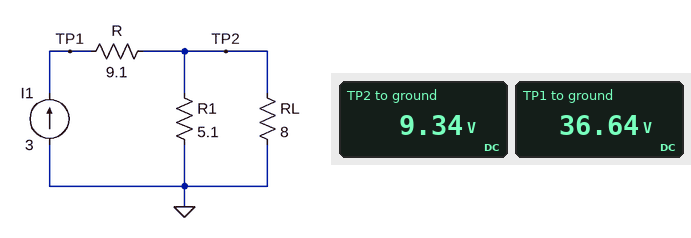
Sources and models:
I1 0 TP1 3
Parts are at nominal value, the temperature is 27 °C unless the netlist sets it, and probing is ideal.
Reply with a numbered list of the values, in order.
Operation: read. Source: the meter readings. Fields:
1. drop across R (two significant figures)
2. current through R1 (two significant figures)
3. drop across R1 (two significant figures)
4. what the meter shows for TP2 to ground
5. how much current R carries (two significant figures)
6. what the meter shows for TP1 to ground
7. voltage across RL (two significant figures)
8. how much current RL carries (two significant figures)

1. 27 V
2. 1.8 A
3. 9.3 V
4. 9.34 V
5. 3.0 A
6. 36.64 V
7. 9.3 V
8. 1.2 A
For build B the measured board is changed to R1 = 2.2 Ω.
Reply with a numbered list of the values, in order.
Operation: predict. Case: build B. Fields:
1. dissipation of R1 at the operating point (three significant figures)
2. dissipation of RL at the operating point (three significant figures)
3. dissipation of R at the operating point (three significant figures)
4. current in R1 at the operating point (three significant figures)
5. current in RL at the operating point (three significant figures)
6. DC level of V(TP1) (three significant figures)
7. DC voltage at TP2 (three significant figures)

1. 12.2 W
2. 3.35 W
3. 81.9 W
4. 2.35 A
5. 647 mA
6. 32.5 V
7. 5.18 V
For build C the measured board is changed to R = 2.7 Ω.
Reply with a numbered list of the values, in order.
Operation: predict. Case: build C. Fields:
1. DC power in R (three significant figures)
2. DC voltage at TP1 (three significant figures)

1. 24.3 W
2. 17.4 V
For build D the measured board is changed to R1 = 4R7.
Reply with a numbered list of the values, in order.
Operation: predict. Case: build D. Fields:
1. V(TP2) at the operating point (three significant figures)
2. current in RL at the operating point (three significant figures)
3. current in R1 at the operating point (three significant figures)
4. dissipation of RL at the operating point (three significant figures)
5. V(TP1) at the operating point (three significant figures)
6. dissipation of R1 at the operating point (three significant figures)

1. 8.88 V
2. 1.11 A
3. 1.89 A
4. 9.86 W
5. 36.2 V
6. 16.8 W
